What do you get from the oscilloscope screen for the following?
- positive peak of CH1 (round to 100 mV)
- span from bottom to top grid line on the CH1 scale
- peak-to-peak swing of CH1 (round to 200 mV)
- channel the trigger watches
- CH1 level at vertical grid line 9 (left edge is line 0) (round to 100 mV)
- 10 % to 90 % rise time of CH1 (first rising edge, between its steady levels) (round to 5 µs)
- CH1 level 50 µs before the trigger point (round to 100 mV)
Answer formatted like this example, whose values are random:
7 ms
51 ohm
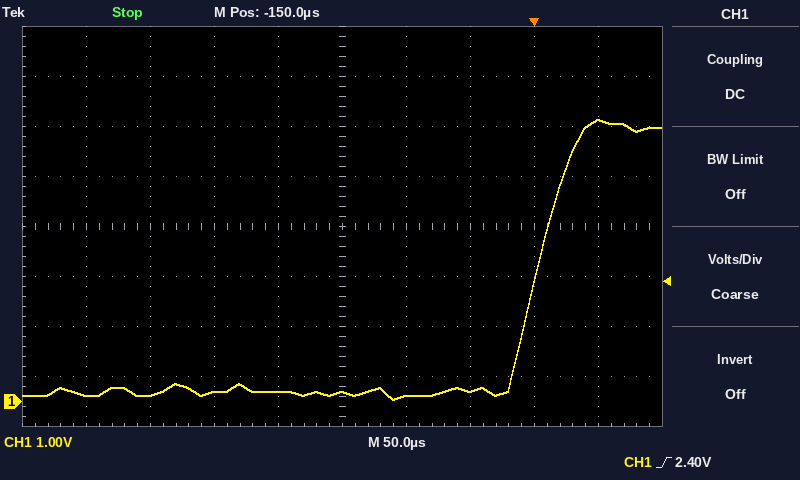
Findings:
5.6 V
8 V
5.6 V
CH1
5.6 V
45 µs
200 mV
